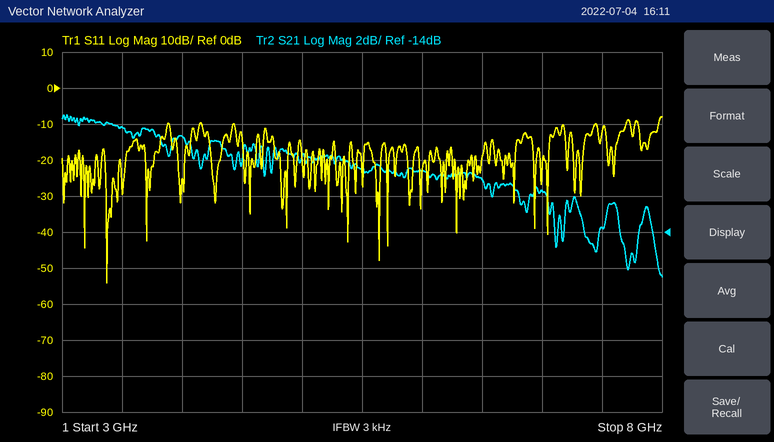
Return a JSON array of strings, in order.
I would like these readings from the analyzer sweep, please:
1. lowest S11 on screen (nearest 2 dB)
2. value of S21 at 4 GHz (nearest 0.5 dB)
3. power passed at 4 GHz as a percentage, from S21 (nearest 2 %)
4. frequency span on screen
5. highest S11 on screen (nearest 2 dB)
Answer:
["-54 dB", "-8.5 dB", "14 %", "5 GHz", "-8 dB"]
